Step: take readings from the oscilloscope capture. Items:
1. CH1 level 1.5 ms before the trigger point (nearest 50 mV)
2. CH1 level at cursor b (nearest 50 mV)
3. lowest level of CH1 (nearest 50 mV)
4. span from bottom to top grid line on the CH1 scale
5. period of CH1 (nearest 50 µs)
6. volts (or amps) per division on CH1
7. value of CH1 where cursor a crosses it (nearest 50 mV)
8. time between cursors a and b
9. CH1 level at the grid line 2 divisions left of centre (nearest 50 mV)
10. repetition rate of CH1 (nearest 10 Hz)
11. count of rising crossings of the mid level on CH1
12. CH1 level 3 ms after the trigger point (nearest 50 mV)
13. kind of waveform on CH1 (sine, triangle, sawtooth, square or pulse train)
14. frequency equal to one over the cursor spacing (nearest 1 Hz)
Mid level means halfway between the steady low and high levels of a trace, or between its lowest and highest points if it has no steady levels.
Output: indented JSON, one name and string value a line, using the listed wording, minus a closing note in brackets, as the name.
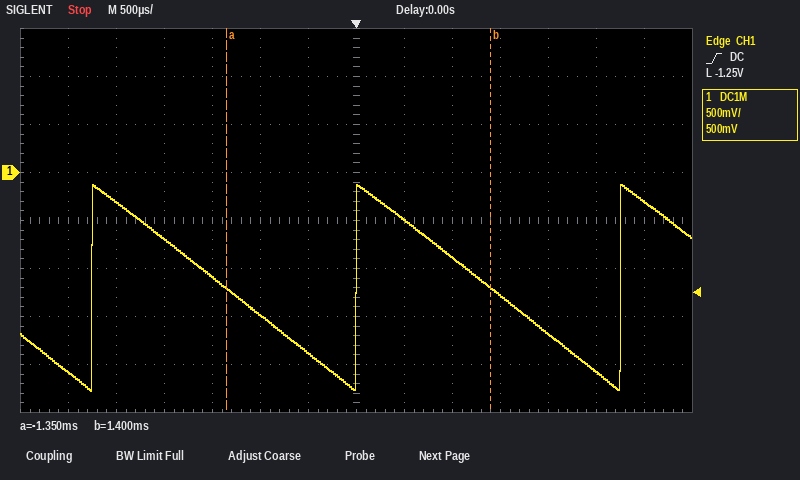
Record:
{
  "CH1 level 1.5 ms before the trigger point": "-1.10 V",
  "CH1 level at cursor b": "-1.20 V",
  "lowest level of CH1": "-2.25 V",
  "span from bottom to top grid line on the CH1 scale": "4 V",
  "period of CH1": "2.75 ms",
  "volts (or amps) per division on CH1": "500 mV",
  "value of CH1 where cursor a crosses it": "-1.20 V",
  "time between cursors a and b": "2.75 ms",
  "CH1 level at the grid line 2 divisions left of centre": "-1.50 V",
  "repetition rate of CH1": "360 Hz",
  "count of rising crossings of the mid level on CH1": "3",
  "CH1 level 3 ms after the trigger point": "-300 mV",
  "kind of waveform on CH1": "sawtooth",
  "frequency equal to one over the cursor spacing": "364 Hz"
}
